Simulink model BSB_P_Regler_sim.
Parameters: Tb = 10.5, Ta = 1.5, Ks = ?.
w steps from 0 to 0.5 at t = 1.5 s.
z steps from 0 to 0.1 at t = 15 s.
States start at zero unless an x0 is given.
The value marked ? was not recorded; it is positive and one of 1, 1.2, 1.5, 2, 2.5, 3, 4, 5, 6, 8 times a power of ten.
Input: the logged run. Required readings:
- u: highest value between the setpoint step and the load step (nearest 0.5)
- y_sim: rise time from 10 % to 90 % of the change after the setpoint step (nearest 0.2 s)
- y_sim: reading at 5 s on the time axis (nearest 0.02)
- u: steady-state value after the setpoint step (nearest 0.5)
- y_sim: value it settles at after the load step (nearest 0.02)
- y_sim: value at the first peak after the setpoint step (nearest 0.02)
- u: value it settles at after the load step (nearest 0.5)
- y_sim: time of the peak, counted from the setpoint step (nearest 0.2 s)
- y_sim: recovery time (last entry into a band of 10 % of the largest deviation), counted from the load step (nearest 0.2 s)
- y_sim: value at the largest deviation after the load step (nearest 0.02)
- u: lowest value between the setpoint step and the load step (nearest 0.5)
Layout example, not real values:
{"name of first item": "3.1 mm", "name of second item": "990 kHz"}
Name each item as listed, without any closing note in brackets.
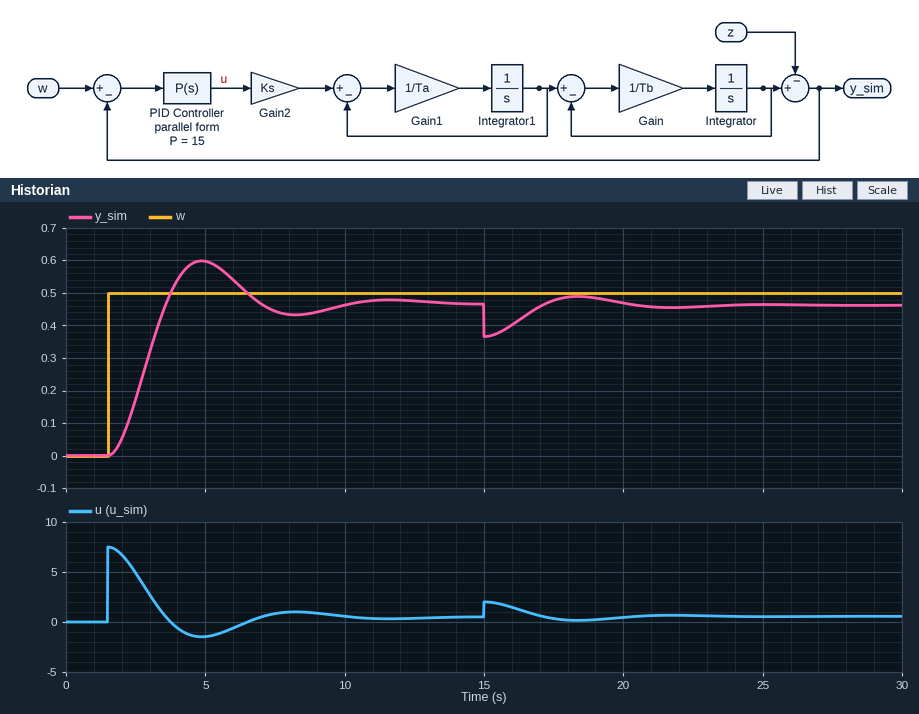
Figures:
{"u: highest value between the setpoint step and the load step": "7.5", "y_sim: rise time from 10 % to 90 % of the change after the setpoint step": "1.4 s", "y_sim: reading at 5 s on the time axis": "0.60", "u: steady-state value after the setpoint step": "0.5", "y_sim: value it settles at after the load step": "0.46", "y_sim: value at the first peak after the setpoint step": "0.60", "u: value it settles at after the load step": "0.5", "y_sim: time of the peak, counted from the setpoint step": "3.4 s", "y_sim: recovery time (last entry into a band of 10 % of the largest deviation), counted from the load step": "4.8 s", "y_sim: value at the largest deviation after the load step": "0.36", "u: lowest value between the setpoint step and the load step": "-1.5"}
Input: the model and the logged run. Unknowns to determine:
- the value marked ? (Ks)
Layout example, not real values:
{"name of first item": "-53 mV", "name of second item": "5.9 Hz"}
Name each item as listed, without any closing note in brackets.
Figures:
{"the value marked ?": "1"}
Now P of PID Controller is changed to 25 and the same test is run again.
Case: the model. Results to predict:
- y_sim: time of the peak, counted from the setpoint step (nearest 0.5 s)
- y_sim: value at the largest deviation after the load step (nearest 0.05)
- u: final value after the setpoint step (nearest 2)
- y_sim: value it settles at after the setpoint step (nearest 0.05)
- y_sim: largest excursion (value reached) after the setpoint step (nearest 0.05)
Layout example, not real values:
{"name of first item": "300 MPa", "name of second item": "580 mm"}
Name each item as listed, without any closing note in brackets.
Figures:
{"y_sim: time of the peak, counted from the setpoint step": "2.5 s", "y_sim: value at the largest deviation after the load step": "0.40", "u: final value after the setpoint step": "0", "y_sim: value it settles at after the setpoint step": "0.50", "y_sim: largest excursion (value reached) after the setpoint step": "0.65"}
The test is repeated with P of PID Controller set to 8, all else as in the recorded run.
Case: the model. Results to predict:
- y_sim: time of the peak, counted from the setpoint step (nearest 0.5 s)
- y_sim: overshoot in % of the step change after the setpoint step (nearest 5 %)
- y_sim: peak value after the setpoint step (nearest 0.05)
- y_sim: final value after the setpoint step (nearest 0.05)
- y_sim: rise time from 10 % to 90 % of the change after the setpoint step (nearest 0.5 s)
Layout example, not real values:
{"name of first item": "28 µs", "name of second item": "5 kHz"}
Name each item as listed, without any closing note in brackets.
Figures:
{"y_sim: time of the peak, counted from the setpoint step": "5.0 s", "y_sim: overshoot in % of the step change after the setpoint step": "15 %", "y_sim: peak value after the setpoint step": "0.50", "y_sim: final value after the setpoint step": "0.45", "y_sim: rise time from 10 % to 90 % of the change after the setpoint step": "2.0 s"}
